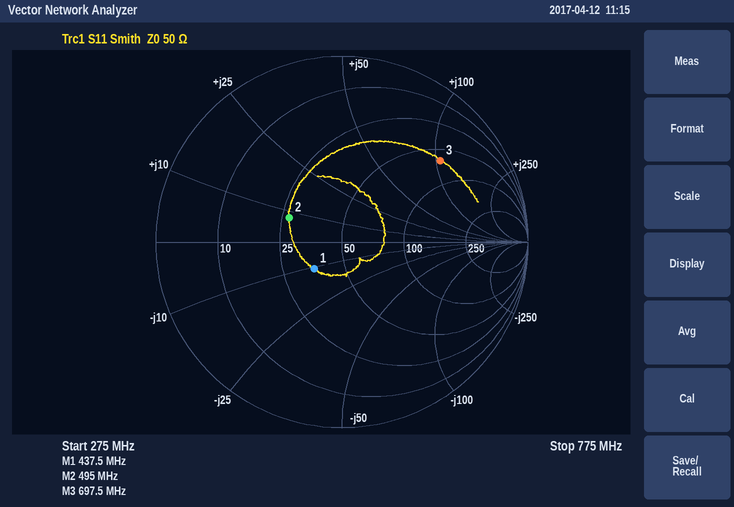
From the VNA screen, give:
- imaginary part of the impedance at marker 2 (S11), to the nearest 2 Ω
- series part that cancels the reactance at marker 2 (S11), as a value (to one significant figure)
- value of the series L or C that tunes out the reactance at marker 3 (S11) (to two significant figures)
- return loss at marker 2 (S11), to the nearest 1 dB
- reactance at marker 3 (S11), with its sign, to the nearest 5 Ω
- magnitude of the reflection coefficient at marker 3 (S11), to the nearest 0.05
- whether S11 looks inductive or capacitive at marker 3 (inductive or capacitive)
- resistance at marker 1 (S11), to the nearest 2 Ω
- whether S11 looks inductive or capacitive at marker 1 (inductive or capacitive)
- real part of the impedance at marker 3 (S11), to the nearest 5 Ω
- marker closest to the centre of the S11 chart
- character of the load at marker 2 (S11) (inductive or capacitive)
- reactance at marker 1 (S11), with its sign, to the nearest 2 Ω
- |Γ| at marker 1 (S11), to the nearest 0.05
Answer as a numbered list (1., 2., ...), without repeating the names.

1. +8 Ω
2. 40 pF
3. 2.2 pF
4. 10 dB
5. +105 Ω
6. 0.70
7. inductive
8. 36 Ω
9. capacitive
10. 65 Ω
11. marker 1
12. inductive
13. -10 Ω
14. 0.20
